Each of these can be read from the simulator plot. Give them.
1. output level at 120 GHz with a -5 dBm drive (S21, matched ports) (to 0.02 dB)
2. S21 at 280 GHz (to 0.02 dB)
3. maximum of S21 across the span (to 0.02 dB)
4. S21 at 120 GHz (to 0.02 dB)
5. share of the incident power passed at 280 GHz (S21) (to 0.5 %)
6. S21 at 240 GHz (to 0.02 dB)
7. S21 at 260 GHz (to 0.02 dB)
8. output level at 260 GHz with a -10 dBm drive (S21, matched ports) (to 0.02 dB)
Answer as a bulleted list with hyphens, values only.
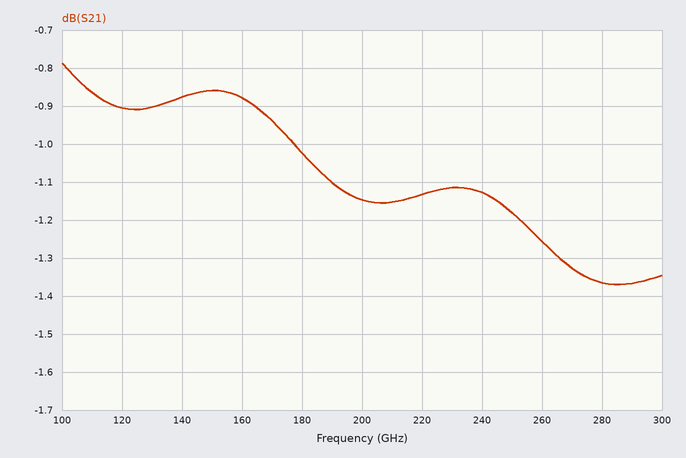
- -5.90 dBm
- -1.36 dB
- -0.78 dB
- -0.90 dB
- 73.0 %
- -1.12 dB
- -1.26 dB
- -11.26 dBm
